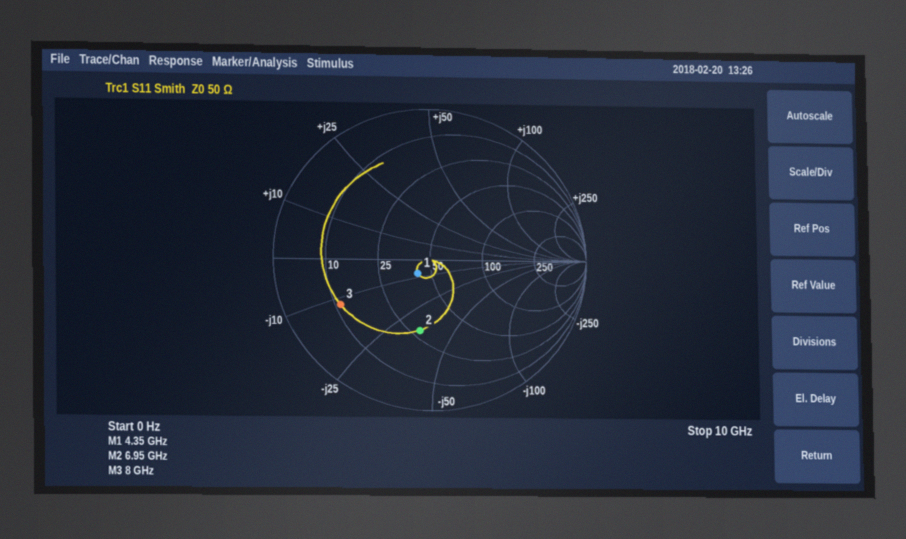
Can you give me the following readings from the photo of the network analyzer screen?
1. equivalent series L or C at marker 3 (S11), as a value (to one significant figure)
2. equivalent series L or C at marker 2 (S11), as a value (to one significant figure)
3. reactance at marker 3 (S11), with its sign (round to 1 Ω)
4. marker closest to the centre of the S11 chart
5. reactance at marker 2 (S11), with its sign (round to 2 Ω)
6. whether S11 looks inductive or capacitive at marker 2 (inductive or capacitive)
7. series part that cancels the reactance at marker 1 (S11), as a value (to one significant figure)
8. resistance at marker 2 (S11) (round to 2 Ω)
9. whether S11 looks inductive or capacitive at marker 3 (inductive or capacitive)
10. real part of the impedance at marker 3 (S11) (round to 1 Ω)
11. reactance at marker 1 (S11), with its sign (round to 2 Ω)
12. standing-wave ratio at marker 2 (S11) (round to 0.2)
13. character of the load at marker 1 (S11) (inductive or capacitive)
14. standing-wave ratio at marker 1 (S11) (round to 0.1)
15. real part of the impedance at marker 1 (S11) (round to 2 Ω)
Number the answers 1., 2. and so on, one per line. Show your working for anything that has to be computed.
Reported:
1. C = 1/(2π × 8 GHz × 12 Ω) ≈ 2 pF
2. C = 1/(2π × 6.95 GHz × 34 Ω) ≈ 674 fF, so 700 fF to one significant figure
3. -12 Ω
4. marker 1
5. -34 Ω
6. capacitive
7. L = 8 Ω/(2π × 4.35 GHz) ≈ 293 pH, so 300 pH to one significant figure
8. 28 Ω
9. capacitive
10. 11 Ω
11. -8 Ω
12. 2.8
13. capacitive
14. 1.3
15. 42 Ω
